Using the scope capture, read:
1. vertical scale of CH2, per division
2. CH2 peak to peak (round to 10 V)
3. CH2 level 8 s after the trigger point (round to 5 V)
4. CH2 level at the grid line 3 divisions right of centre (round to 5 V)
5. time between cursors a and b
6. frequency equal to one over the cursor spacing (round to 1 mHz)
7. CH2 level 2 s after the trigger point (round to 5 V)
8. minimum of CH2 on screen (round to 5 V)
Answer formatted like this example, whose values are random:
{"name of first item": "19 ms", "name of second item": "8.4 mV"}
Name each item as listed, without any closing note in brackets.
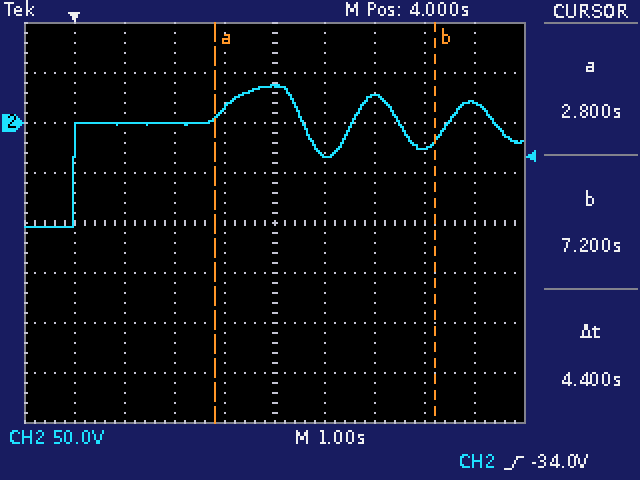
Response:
{"vertical scale of CH2, per division": "50 V", "CH2 peak to peak": "140 V", "CH2 level 8 s after the trigger point": "20 V", "CH2 level at the grid line 3 divisions right of centre": "-25 V", "time between cursors a and b": "4.4 s", "frequency equal to one over the cursor spacing": "227 mHz", "CH2 level 2 s after the trigger point": "0 V", "minimum of CH2 on screen": "-105 V"}
